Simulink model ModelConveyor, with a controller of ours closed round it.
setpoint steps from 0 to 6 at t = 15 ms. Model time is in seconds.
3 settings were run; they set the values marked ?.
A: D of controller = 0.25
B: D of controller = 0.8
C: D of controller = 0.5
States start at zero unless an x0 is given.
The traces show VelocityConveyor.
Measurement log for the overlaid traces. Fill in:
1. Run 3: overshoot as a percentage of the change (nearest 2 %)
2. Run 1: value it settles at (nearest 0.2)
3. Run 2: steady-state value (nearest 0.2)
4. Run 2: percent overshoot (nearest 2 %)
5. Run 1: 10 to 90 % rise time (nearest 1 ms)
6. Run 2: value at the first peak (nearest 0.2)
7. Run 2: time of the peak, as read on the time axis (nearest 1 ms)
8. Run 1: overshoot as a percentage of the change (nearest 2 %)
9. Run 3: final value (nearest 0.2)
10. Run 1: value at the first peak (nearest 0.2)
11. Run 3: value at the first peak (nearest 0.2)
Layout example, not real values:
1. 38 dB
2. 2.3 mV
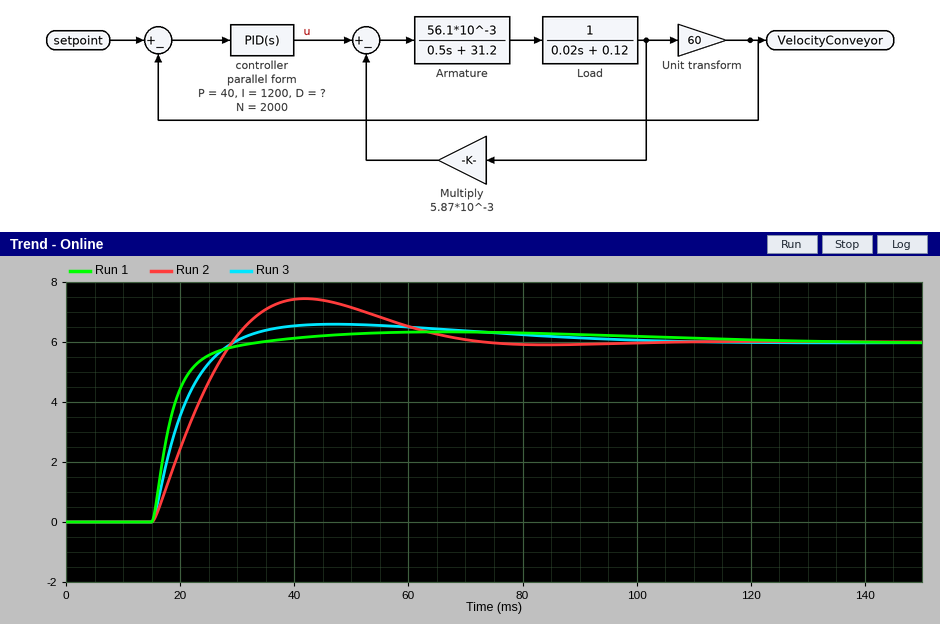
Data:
1. 10 %
2. 6.0
3. 6.0
4. 24 %
5. 8 ms
6. 7.4
7. 42 ms
8. 6 %
9. 6.0
10. 6.4
11. 6.6
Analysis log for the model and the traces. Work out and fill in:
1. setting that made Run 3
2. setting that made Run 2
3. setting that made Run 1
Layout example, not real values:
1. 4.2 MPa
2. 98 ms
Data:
1. C
2. A
3. B
